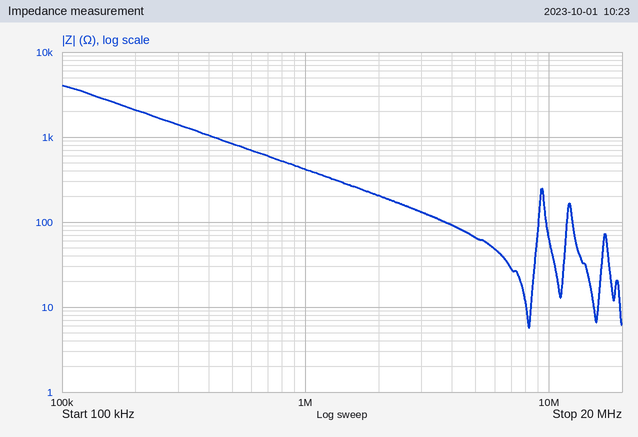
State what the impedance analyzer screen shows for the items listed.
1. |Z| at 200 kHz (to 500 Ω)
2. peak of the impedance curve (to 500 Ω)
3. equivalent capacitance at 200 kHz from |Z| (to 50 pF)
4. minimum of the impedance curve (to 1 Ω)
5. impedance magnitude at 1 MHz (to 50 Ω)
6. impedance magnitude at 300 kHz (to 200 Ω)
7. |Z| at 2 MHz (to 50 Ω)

2.0 kΩ
4.0 kΩ
400 pF
6 Ω
400 Ω
1.4 kΩ
200 Ω
